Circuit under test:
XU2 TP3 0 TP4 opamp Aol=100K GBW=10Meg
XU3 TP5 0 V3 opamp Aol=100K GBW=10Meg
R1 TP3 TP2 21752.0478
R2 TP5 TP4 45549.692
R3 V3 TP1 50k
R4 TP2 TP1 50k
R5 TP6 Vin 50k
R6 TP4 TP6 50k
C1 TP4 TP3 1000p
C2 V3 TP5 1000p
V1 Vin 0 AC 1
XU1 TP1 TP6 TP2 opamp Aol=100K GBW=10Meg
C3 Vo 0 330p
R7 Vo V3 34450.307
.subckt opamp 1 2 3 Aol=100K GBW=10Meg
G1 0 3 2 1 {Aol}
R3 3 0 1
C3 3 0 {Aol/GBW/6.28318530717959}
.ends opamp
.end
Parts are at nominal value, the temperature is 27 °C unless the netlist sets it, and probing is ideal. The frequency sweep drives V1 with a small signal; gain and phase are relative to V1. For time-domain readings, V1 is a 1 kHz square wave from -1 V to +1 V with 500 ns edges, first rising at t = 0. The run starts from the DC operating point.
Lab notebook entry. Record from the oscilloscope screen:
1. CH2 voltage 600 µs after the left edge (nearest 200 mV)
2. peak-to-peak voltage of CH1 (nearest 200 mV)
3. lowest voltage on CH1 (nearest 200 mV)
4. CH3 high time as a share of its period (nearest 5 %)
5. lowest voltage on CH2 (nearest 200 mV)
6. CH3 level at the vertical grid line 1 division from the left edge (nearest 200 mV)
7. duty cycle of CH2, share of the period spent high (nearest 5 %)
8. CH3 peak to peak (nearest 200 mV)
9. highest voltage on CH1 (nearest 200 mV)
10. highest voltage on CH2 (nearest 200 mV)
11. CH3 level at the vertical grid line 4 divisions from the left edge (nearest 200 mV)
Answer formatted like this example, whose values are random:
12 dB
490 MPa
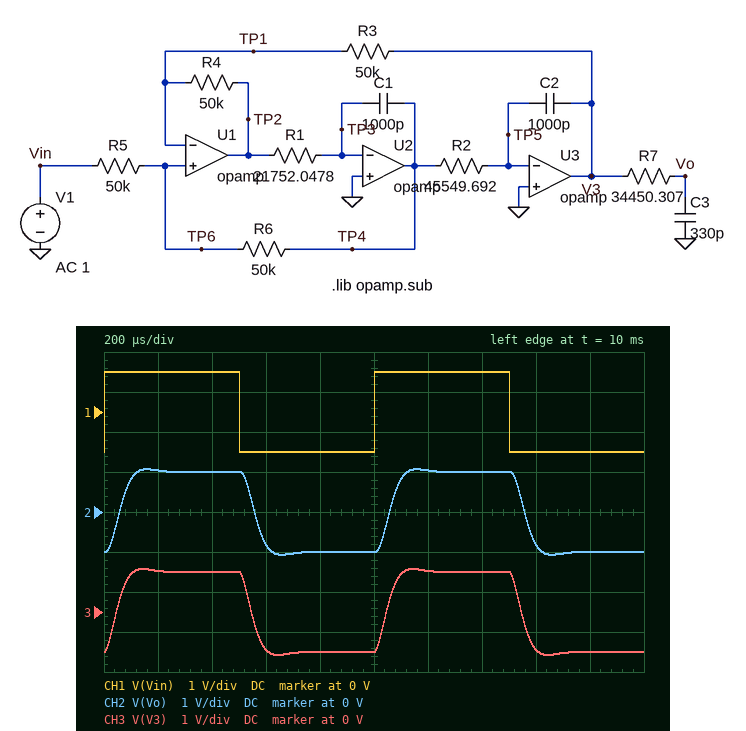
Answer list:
-800 mV
2.0 V
-1.0 V
50 %
-1.0 V
1.0 V
50 %
2.2 V
1.0 V
1.0 V
-1.0 V
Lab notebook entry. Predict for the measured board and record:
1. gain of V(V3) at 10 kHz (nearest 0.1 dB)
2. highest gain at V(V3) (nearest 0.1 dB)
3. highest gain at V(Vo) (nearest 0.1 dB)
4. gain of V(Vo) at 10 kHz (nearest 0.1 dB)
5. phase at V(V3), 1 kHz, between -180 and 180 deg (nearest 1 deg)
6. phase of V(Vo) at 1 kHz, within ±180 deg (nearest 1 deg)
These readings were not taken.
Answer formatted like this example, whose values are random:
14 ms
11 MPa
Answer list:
-12.2 dB
0 dB
0 dB
-14.0 dB
-17 deg
-21 deg
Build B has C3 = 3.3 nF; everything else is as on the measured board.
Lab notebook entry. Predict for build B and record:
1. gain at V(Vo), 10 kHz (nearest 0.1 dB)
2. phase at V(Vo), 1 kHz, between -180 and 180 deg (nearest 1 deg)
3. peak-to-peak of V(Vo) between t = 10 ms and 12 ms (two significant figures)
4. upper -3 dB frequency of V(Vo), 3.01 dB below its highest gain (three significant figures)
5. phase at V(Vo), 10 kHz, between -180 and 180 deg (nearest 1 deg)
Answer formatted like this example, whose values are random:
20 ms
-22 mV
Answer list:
-29.4 dB
-52 deg
1.9 V
1.38 kHz
142 deg
